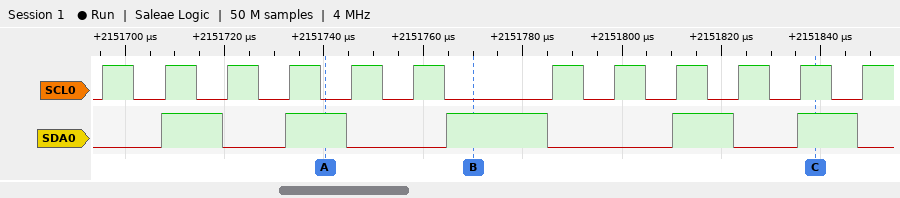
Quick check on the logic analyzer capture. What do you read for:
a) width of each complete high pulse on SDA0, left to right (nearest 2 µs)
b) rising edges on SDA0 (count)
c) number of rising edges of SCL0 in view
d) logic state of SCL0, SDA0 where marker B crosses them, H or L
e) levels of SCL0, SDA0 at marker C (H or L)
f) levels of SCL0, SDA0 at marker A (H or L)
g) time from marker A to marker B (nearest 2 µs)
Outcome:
12 µs, 12 µs, 20 µs, 12 µs, 12 µs
5
12
SCL0=L, SDA0=H
SCL0=H, SDA0=H
SCL0=L, SDA0=H
30 µs
